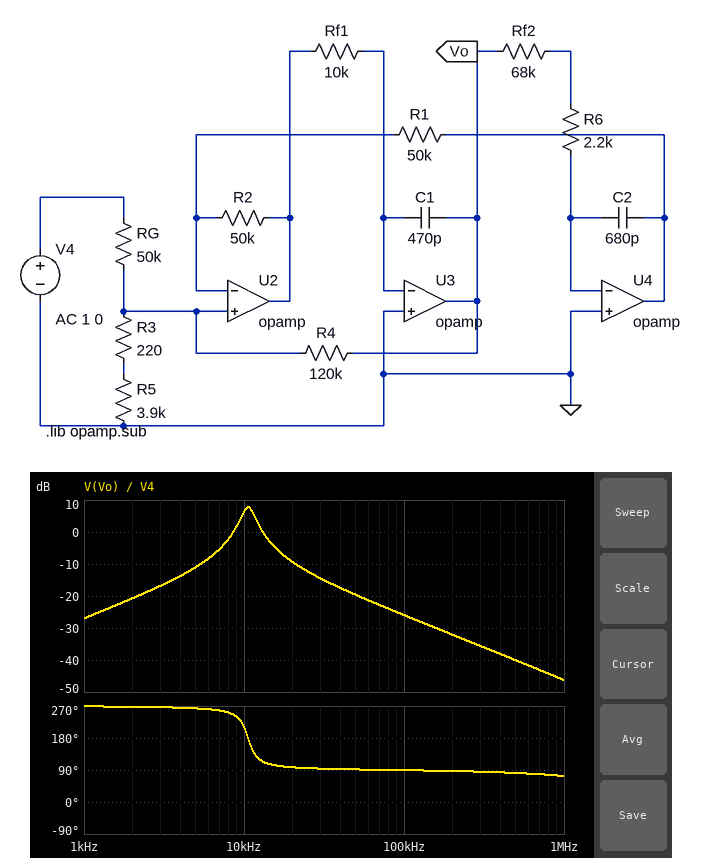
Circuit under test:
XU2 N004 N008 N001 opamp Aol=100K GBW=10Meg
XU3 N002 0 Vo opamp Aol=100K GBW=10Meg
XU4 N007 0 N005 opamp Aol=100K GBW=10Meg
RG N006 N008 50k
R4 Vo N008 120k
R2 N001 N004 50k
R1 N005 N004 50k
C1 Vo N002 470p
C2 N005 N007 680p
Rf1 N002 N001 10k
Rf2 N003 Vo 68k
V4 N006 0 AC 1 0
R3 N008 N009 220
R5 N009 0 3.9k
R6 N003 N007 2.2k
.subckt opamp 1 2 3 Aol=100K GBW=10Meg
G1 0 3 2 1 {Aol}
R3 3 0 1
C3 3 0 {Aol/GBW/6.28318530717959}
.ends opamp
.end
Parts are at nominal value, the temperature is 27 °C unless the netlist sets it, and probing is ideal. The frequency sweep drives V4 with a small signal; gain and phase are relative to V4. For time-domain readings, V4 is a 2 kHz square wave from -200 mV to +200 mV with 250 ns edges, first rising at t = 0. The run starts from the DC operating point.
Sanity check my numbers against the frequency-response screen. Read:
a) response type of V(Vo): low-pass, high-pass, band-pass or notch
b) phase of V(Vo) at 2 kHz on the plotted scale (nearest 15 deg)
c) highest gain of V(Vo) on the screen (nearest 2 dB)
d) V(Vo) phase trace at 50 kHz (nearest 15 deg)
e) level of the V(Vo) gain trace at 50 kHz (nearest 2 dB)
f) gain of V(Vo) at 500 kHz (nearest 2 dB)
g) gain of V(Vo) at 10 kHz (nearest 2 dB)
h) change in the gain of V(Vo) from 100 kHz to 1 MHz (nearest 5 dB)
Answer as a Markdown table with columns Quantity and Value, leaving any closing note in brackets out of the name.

| Quantity | Value |
|---|---|
| response type of V(Vo): low-pass, high-pass, band-pass or notch | band-pass |
| phase of V(Vo) at 2 kHz on the plotted scale | 270 deg |
| highest gain of V(Vo) on the screen | 8 dB |
| V(Vo) phase trace at 50 kHz | 90 deg |
| level of the V(Vo) gain trace at 50 kHz | -20 dB |
| gain of V(Vo) at 500 kHz | -40 dB |
| gain of V(Vo) at 10 kHz | 6 dB |
| change in the gain of V(Vo) from 100 kHz to 1 MHz | -20 dB |
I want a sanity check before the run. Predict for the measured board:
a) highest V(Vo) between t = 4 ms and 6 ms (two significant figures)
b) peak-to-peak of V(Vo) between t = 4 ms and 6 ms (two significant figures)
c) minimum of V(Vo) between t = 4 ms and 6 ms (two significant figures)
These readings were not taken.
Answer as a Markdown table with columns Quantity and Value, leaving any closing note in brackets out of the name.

| Quantity | Value |
|---|---|
| highest V(Vo) between t = 4 ms and 6 ms | 190 mV |
| peak-to-peak of V(Vo) between t = 4 ms and 6 ms | 380 mV |
| minimum of V(Vo) between t = 4 ms and 6 ms | -190 mV |
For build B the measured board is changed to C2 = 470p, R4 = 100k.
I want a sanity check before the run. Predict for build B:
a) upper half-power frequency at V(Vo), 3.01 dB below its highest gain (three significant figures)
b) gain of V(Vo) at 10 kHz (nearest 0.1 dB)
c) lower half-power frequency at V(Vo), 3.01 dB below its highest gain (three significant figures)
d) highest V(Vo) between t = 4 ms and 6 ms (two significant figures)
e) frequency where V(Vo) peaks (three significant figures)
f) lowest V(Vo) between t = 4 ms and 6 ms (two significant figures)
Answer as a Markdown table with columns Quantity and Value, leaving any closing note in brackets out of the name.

| Quantity | Value |
|---|---|
| upper half-power frequency at V(Vo), 3.01 dB below its highest gain | 14.0 kHz |
| gain of V(Vo) at 10 kHz | -2.7 dB |
| lower half-power frequency at V(Vo), 3.01 dB below its highest gain | 11.6 kHz |
| highest V(Vo) between t = 4 ms and 6 ms | 120 mV |
| frequency where V(Vo) peaks | 12.8 kHz |
| lowest V(Vo) between t = 4 ms and 6 ms | -120 mV |
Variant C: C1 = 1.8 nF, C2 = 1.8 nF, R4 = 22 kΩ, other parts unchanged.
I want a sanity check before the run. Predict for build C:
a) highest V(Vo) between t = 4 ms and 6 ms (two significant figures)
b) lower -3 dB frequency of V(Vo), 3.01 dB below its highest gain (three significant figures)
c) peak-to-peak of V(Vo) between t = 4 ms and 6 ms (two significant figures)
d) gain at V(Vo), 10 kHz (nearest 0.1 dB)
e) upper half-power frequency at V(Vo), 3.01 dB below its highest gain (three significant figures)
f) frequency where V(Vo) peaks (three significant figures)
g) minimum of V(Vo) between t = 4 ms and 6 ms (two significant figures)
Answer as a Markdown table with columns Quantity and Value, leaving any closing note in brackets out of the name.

| Quantity | Value |
|---|---|
| highest V(Vo) between t = 4 ms and 6 ms | 86 mV |
| lower -3 dB frequency of V(Vo), 3.01 dB below its highest gain | 2.28 kHz |
| peak-to-peak of V(Vo) between t = 4 ms and 6 ms | 170 mV |
| gain at V(Vo), 10 kHz | -18.1 dB |
| upper half-power frequency at V(Vo), 3.01 dB below its highest gain | 4.88 kHz |
| frequency where V(Vo) peaks | 3.34 kHz |
| minimum of V(Vo) between t = 4 ms and 6 ms | -86 mV |
